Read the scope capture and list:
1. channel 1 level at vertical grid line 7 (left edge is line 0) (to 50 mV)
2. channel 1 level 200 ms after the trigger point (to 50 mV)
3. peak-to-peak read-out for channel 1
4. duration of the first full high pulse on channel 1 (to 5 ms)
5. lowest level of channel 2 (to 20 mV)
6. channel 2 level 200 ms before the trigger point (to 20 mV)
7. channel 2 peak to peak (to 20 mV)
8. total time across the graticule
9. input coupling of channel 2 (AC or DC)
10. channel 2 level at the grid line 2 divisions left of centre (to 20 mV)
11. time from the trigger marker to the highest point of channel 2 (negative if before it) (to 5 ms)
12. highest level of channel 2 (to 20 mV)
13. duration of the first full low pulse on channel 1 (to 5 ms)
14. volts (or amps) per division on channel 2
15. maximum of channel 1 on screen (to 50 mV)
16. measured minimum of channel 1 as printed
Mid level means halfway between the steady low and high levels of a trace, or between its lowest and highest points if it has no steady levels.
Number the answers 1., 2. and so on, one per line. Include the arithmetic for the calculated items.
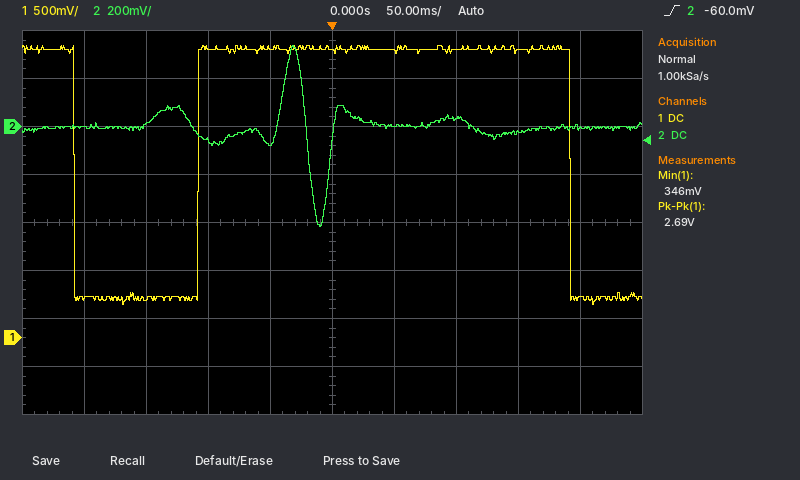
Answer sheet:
1. 3.00 V
2. 400 mV
3. 2.69 V
4. 300 ms
5. -420 mV
6. 0 mV
7. 340 mV − (-420 mV) = 760 mV
8. 500 ms
9. DC
10. -60 mV
11. -30 ms
12. 340 mV
13. 100 ms
14. 200 mV
15. 3.05 V
16. 346 mV
